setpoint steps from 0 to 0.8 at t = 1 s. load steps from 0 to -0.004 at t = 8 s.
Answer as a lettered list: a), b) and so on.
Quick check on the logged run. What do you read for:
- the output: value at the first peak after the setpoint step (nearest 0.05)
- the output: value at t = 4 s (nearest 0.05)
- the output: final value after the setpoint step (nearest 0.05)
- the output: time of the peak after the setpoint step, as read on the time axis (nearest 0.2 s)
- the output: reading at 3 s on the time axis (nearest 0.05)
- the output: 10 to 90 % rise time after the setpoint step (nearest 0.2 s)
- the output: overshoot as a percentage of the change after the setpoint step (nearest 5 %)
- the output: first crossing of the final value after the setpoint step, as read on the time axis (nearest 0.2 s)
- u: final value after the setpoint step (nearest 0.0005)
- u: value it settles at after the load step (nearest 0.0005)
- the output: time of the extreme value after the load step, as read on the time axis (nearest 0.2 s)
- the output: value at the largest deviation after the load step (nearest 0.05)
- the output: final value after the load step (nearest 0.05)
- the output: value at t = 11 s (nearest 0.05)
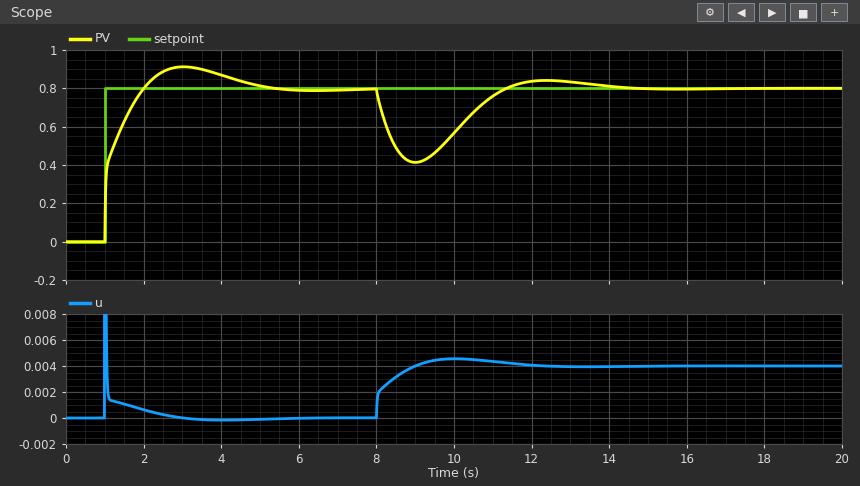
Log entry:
a) 0.90
b) 0.85
c) 0.80
d) 3.0 s
e) 0.90
f) 0.8 s
g) 15 %
h) 2.0 s
i) 0.0000
j) 0.0040
k) 9.0 s
l) 0.40
m) 0.80
n) 0.75
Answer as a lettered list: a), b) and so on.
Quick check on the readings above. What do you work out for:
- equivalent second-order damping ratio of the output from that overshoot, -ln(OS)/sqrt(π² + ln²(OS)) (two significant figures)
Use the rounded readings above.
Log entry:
a) 0.52
